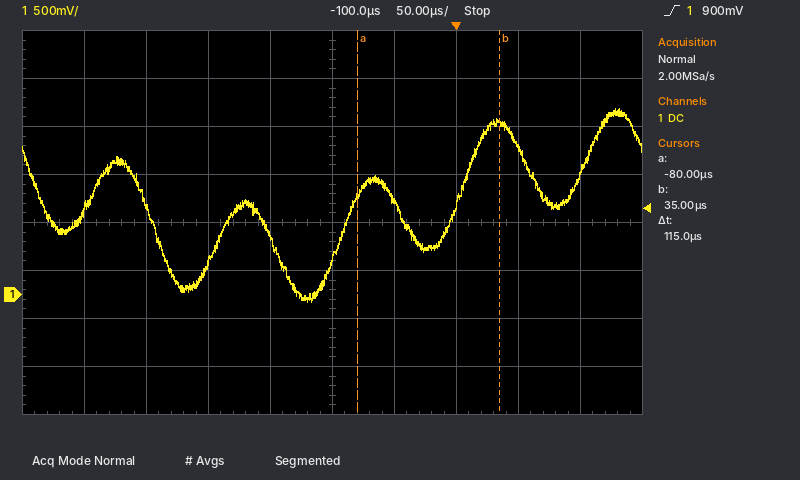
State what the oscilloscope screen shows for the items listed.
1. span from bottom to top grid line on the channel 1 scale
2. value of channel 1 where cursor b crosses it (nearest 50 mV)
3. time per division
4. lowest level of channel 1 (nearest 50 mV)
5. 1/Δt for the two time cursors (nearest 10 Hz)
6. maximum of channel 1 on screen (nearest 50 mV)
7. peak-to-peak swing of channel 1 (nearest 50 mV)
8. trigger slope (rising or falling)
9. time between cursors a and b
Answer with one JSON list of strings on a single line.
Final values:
["4 V", "1.80 V", "50 µs", "-50 mV", "8.70 kHz", "1.95 V", "2.00 V", "rising", "115 µs"]
